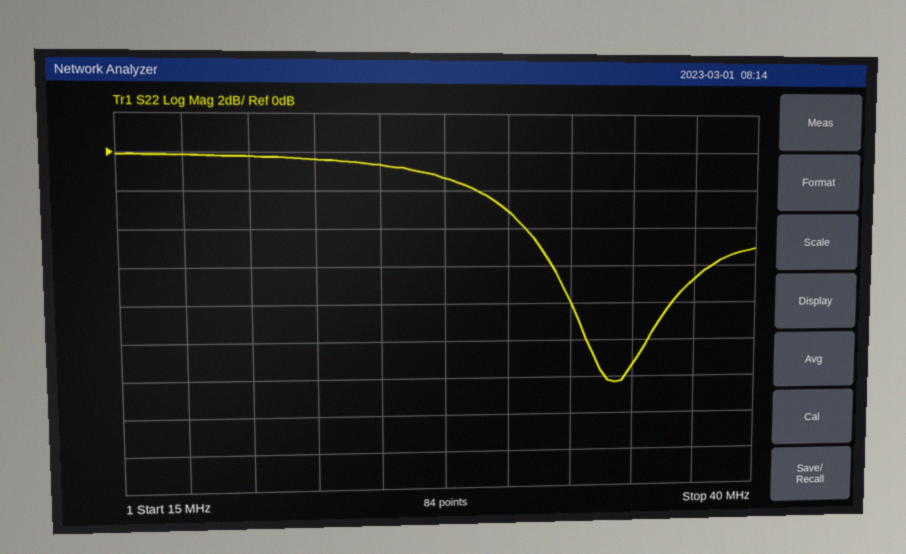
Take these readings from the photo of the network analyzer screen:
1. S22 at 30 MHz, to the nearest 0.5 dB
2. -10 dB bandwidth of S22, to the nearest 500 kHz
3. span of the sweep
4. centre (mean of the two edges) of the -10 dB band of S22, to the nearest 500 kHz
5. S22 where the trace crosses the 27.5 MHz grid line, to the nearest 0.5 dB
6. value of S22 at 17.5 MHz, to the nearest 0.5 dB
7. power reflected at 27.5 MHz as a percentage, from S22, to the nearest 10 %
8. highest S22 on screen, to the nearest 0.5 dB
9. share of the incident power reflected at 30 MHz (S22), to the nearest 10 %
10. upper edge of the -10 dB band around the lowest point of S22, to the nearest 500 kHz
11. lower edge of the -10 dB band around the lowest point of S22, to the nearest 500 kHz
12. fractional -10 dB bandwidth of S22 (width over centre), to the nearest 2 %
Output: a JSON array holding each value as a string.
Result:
["-3.0 dB", "2.5 MHz", "25 MHz", "34.5 MHz", "-1.5 dB", "0.0 dB", "70 %", "0.0 dB", "50 %", "35.5 MHz", "33.0 MHz", "8 %"]
